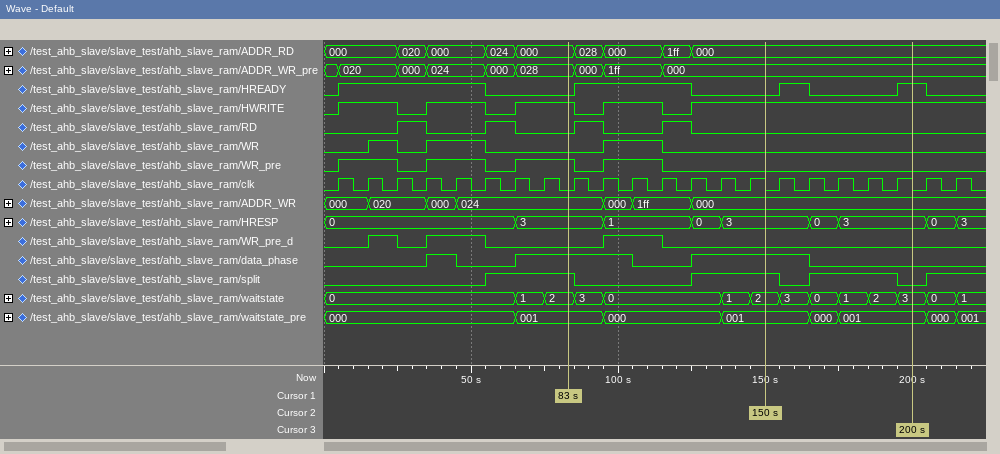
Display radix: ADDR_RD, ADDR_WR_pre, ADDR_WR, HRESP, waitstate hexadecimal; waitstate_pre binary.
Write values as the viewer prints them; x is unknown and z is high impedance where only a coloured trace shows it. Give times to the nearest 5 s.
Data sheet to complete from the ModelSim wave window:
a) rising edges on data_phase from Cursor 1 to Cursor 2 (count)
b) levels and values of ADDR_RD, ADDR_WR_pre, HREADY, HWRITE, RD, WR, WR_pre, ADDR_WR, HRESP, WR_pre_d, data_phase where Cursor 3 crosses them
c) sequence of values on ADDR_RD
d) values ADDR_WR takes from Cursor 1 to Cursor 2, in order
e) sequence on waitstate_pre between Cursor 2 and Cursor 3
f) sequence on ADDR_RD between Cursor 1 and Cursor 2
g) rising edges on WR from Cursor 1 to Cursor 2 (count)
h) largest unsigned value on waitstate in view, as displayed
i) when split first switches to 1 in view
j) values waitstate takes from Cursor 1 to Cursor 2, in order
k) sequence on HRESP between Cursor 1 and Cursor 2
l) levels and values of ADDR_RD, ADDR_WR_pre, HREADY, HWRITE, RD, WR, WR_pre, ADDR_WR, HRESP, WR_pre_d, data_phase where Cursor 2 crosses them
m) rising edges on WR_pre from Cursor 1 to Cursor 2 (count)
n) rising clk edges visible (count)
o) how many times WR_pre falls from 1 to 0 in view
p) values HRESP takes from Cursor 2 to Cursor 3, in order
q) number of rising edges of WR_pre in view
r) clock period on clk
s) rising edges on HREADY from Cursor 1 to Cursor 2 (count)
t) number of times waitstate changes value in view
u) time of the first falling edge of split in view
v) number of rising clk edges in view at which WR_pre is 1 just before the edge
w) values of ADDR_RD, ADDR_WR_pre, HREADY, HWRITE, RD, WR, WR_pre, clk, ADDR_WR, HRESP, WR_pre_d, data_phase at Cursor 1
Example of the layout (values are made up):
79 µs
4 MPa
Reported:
1
ADDR_RD=000, ADDR_WR_pre=000, HREADY=1, HWRITE=1, RD=0, WR=0, WR_pre=0, ADDR_WR=000, HRESP=3, WR_pre_d=0, data_phase=0
000, 020, 000, 024, 000, 028, 000, 1ff, 000
024, 000, 1ff, 000
001, 000, 001
000, 028, 000, 1ff, 000
1
3
55 s
2, 3, 0, 1, 2
3, 1, 0, 3
ADDR_RD=000, ADDR_WR_pre=000, HREADY=0, HWRITE=1, RD=0, WR=0, WR_pre=0, ADDR_WR=000, HRESP=3, WR_pre_d=0, data_phase=1
1
22
4
3, 0, 3
4
10 s
1
13
85 s
8
ADDR_RD=000, ADDR_WR_pre=028, HREADY=0, HWRITE=1, RD=0, WR=0, WR_pre=1, clk=0, ADDR_WR=024, HRESP=3, WR_pre_d=0, data_phase=1
